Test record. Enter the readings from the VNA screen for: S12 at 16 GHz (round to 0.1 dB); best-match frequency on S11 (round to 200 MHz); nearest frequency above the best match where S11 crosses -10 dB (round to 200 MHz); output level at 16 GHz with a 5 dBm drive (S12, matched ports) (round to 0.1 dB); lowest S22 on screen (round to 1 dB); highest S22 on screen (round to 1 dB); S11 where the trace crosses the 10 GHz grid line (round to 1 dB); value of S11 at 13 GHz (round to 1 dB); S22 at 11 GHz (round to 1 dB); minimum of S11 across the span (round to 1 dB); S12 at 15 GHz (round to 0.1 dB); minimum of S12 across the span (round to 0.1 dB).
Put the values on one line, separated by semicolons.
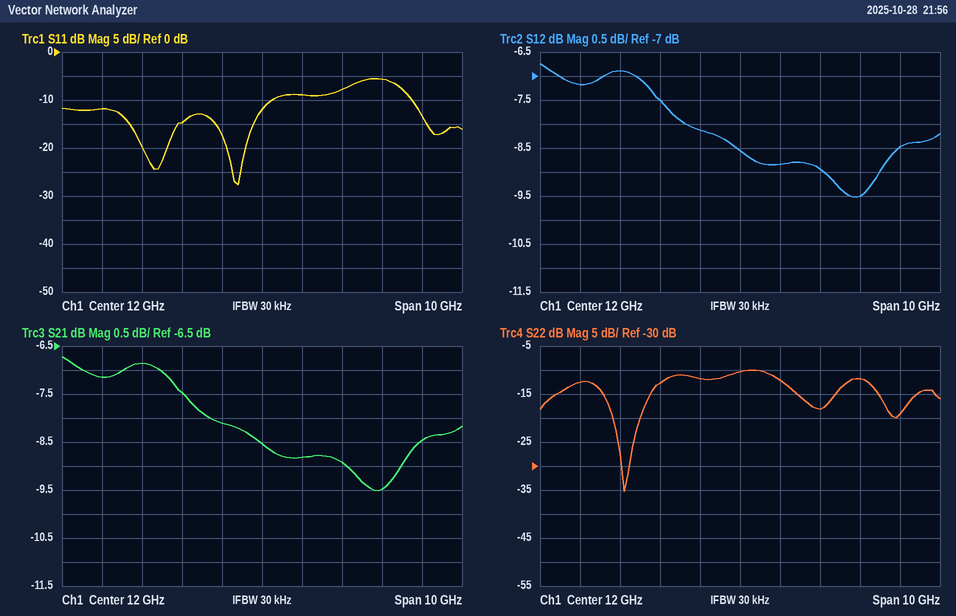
-8.5 dB; 11.4 GHz; 12.2 GHz; -3.5 dBm; -35 dB; -10 dB; -15 dB; -9 dB; -12 dB; -28 dB; -9.5 dB; -9.5 dB
